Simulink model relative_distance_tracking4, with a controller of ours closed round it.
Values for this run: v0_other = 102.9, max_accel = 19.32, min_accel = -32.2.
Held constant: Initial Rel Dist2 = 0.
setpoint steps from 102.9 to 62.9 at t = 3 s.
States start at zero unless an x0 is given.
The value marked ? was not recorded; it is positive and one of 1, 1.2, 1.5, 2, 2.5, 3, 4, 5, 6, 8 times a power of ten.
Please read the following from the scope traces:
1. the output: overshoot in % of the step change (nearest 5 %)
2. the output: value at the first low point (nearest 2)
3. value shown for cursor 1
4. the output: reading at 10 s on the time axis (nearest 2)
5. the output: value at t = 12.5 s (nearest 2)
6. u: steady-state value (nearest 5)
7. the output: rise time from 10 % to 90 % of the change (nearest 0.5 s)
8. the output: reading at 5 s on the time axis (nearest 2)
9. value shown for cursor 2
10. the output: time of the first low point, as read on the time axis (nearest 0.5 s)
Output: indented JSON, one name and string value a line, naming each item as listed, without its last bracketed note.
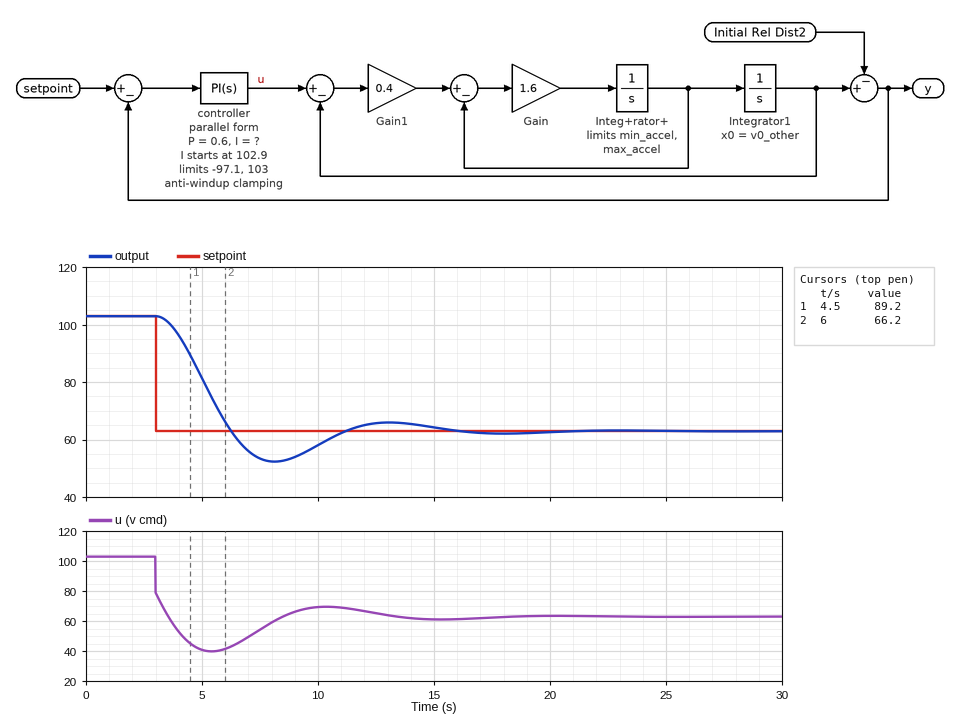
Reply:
{
  "the output: overshoot in % of the step change": "25 %",
  "the output: value at the first low point": "52",
  "value shown for cursor 1": "89.2",
  "the output: reading at 10 s on the time axis": "58",
  "the output: value at t = 12.5 s": "66",
  "u: steady-state value": "65",
  "the output: rise time from 10 % to 90 % of the change": "2.0 s",
  "the output: reading at 5 s on the time axis": "82",
  "value shown for cursor 2": "66.2",
  "the output: time of the first low point, as read on the time axis": "8.0 s"
}
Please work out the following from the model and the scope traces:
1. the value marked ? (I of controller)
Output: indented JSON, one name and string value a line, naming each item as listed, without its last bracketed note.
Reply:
{
  "the value marked ?": "0.8"
}
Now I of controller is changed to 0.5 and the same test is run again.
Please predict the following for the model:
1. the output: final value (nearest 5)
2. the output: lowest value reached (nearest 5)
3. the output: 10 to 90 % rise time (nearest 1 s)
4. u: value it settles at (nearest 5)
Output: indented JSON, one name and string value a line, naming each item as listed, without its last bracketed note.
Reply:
{
  "the output: final value": "65",
  "the output: lowest value reached": "60",
  "the output: 10 to 90 % rise time": "3 s",
  "u: value it settles at": "65"
}
